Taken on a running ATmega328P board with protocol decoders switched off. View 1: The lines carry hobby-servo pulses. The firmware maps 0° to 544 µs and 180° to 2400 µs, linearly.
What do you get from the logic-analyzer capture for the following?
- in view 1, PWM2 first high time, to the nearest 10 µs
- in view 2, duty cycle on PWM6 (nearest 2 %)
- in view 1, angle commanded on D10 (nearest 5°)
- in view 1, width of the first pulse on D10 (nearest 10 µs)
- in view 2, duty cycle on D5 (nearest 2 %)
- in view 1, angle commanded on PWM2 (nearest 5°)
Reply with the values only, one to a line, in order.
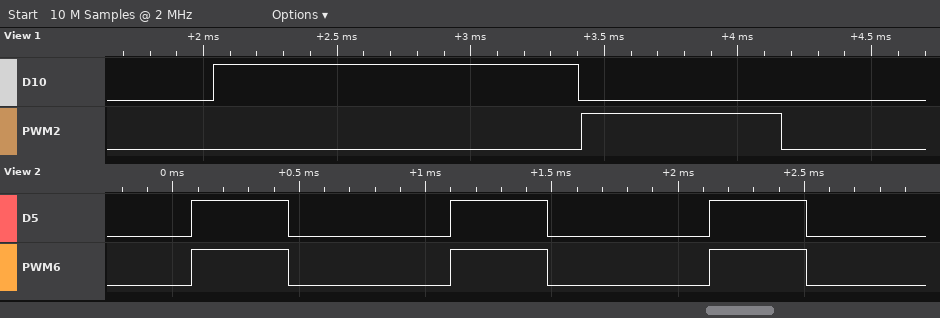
750 µs
38 %
80°
1370 µs
38 %
20°
